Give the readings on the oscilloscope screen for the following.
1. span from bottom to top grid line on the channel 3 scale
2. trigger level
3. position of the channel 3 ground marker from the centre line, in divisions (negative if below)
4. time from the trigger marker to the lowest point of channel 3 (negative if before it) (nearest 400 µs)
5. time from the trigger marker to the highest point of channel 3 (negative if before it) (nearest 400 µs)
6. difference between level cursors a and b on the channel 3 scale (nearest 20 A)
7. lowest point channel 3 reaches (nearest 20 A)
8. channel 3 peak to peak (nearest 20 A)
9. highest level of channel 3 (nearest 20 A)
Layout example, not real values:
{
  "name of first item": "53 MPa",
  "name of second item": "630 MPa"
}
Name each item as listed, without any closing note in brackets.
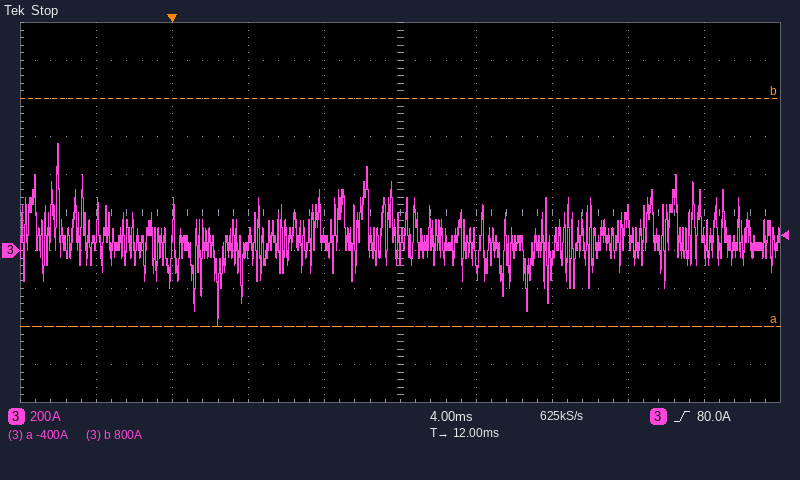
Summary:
{
  "span from bottom to top grid line on the channel 3 scale": "2 kA",
  "trigger level": "80.0 A",
  "position of the channel 3 ground marker from the centre line, in divisions": "-1.0 div",
  "time from the trigger marker to the lowest point of channel 3 (negative if before it)": "+2.4 ms",
  "time from the trigger marker to the highest point of channel 3 (negative if before it)": "-6.0 ms",
  "difference between level cursors a and b on the channel 3 scale": "1.20 kA",
  "lowest point channel 3 reaches": "-400 A",
  "channel 3 peak to peak": "960 A",
  "highest level of channel 3": "560 A"
}
